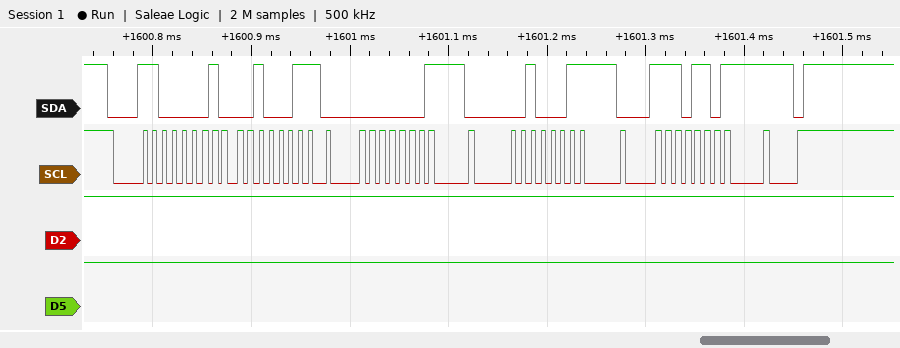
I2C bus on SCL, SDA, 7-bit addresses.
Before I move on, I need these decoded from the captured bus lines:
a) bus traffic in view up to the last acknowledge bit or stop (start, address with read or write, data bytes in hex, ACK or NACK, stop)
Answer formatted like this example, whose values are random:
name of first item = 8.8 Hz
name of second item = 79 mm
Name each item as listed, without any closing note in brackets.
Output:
bus traffic in view up to the last acknowledge bit or stop = start, address 60 read ACK, 23 ACK, 01 ACK, 23 ACK, ED NACK, stop
